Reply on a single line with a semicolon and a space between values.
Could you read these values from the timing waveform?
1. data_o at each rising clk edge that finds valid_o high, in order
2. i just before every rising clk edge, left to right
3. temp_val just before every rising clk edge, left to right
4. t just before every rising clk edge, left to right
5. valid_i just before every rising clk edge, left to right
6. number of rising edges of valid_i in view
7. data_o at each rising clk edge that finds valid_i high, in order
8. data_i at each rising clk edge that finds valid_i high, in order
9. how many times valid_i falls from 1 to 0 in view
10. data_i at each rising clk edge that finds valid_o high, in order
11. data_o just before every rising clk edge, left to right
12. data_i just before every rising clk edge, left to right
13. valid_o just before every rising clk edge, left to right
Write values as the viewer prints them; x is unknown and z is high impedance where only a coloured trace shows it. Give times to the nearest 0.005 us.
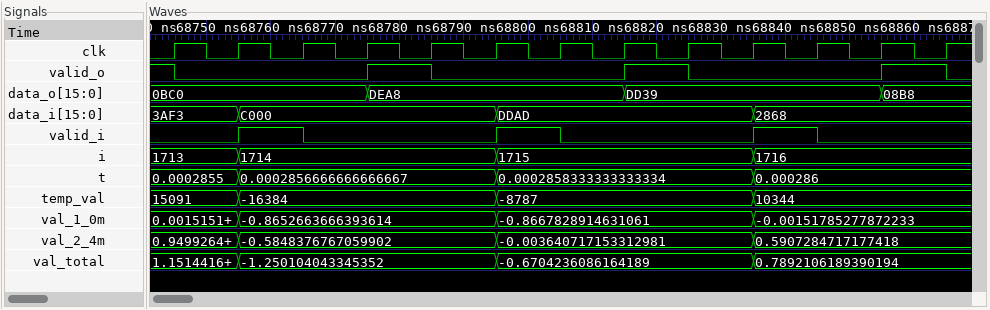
0BC0, DEA8, DD39, 08B8; 1713, 1713, 1714, 1714, 1714, 1714, 1715, 1715, 1715, 1715, 1716, 1716, 1716; 15091, 15091, -16384, -16384, -16384, -16384, -8787, -8787, -8787, -8787, 10344, 10344, 10344; 0.0002855, 0.0002855, 0.0002856666666666667, 0.0002856666666666667, 0.0002856666666666667, 0.0002856666666666667, 0.0002858333333333334, 0.0002858333333333334, 0.0002858333333333334, 0.0002858333333333334, 0.000286, 0.000286, 0.000286; 0 0 1 0 0 0 1 0 0 0 1 0 0; 3; 0BC0, DEA8, DD39; C000, DDAD, 2868; 3; 3AF3, C000, DDAD, 2868; 0BC0, 0BC0, 0BC0, 0BC0, DEA8, DEA8, DEA8, DEA8, DD39, DD39, DD39, DD39, 08B8; 3AF3, 3AF3, C000, C000, C000, C000, DDAD, DDAD, DDAD, DDAD, 2868, 2868, 2868; 1 0 0 0 1 0 0 0 1 0 0 0 1
